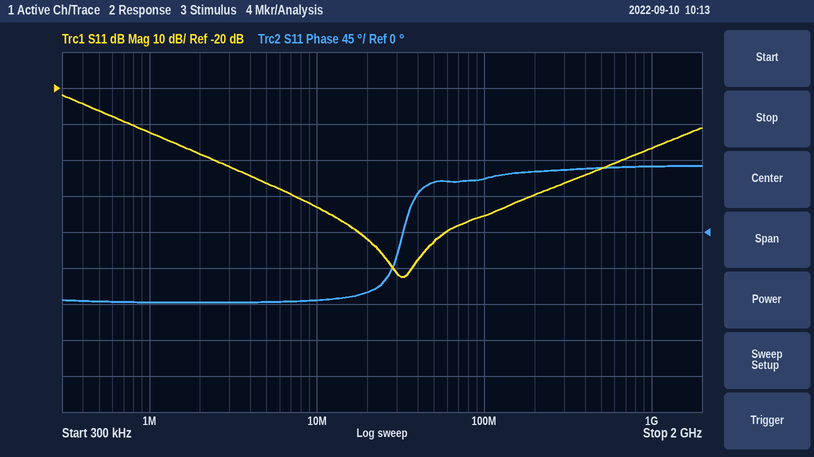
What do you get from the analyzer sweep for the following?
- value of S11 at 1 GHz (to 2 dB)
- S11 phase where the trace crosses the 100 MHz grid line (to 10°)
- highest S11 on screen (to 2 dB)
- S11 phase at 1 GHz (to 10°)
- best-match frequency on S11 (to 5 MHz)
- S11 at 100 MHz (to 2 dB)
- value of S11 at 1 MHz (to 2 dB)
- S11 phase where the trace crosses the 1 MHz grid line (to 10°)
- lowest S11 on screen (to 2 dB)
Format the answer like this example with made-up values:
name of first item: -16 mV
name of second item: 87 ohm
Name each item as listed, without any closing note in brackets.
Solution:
value of S11 at 1 GHz: -36 dB
S11 phase where the trace crosses the 100 MHz grid line: 70°
highest S11 on screen: -22 dB
S11 phase at 1 GHz: 80°
best-match frequency on S11: 30 MHz
S11 at 100 MHz: -56 dB
value of S11 at 1 MHz: -32 dB
S11 phase where the trace crosses the 1 MHz grid line: -90°
lowest S11 on screen: -72 dB
